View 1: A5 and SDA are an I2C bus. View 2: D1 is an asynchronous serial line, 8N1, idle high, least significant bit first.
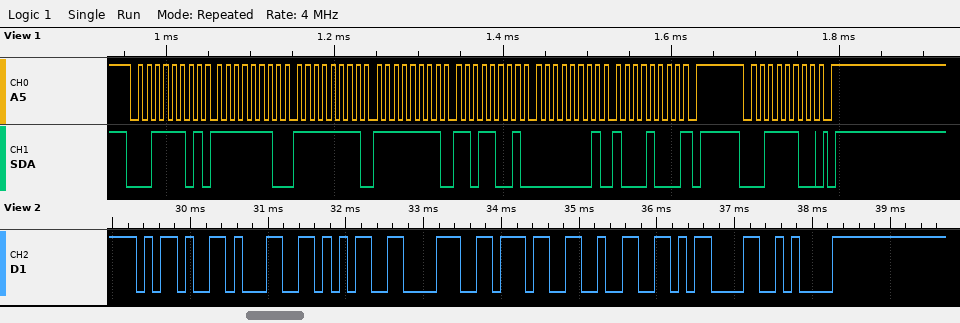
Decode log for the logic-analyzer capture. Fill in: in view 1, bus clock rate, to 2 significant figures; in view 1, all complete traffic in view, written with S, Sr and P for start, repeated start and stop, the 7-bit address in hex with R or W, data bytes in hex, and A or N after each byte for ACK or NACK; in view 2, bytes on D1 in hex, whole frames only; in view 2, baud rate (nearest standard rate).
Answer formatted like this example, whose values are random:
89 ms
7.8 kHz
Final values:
100 kHz
S 1ER A FE A FF A FF A D9 A 01 A 88 N P S 1EW A P
2D 31 35 38 37 32 0D 0A
9600 baud
